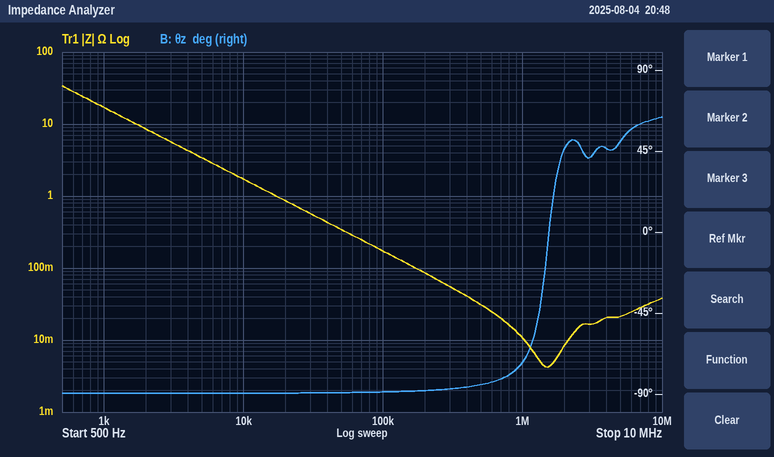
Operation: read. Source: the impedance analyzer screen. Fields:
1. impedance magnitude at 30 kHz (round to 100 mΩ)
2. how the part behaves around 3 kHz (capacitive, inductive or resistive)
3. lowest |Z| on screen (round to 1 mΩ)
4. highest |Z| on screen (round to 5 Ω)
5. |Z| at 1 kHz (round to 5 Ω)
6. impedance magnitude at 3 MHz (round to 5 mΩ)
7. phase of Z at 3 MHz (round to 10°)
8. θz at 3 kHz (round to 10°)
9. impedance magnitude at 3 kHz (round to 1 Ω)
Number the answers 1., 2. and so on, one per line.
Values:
1. 600 mΩ
2. capacitive
3. 4 mΩ
4. 35 Ω
5. 15 Ω
6. 15 mΩ
7. 40°
8. -90°
9. 6 Ω
